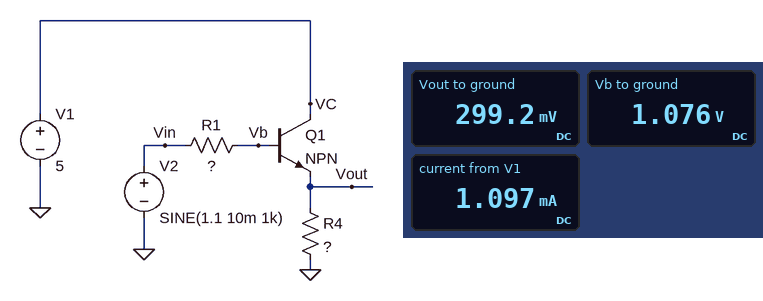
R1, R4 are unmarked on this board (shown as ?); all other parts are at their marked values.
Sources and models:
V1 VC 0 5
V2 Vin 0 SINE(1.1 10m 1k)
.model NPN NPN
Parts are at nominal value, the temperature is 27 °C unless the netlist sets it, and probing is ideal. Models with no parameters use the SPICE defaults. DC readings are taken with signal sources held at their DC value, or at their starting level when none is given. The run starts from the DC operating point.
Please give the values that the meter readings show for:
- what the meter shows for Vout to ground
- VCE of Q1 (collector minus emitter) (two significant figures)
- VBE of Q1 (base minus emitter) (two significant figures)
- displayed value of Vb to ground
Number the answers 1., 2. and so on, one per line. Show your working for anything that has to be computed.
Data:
1. 299.2 mV
2. 5 V - 299.2 mV = 4.7 V
3. 1.076 V - 299.2 mV = 780 mV
4. 1.076 V
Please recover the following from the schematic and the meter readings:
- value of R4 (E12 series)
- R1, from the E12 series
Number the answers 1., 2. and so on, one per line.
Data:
1. 270 Ω
2. 2.2 kΩ
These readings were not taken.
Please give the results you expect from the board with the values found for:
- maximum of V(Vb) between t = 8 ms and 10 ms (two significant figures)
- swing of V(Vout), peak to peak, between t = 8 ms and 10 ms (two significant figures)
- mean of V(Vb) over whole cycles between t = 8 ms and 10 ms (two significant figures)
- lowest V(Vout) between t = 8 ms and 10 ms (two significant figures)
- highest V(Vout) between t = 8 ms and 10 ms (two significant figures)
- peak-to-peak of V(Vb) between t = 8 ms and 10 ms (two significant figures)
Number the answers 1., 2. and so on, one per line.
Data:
1. 1.1 V
2. 17 mV
3. 1.1 V
4. 290 mV
5. 310 mV
6. 19 mV
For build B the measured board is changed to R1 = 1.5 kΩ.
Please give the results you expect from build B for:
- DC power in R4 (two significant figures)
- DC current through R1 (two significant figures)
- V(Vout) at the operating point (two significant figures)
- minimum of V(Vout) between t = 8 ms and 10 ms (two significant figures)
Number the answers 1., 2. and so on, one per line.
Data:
1. 350 µW
2. 11 µA
3. 310 mV
4. 300 mV
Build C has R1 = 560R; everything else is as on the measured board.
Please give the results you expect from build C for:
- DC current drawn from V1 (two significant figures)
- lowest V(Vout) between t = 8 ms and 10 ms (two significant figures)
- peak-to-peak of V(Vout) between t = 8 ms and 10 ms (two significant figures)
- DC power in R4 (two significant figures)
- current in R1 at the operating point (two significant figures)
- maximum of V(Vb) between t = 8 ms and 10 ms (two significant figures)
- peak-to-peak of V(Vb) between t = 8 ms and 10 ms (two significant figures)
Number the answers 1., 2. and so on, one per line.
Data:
1. 1.2 mA
2. 310 mV
3. 18 mV
4. 370 µW
5. 12 µA
6. 1.1 V
7. 20 mV
